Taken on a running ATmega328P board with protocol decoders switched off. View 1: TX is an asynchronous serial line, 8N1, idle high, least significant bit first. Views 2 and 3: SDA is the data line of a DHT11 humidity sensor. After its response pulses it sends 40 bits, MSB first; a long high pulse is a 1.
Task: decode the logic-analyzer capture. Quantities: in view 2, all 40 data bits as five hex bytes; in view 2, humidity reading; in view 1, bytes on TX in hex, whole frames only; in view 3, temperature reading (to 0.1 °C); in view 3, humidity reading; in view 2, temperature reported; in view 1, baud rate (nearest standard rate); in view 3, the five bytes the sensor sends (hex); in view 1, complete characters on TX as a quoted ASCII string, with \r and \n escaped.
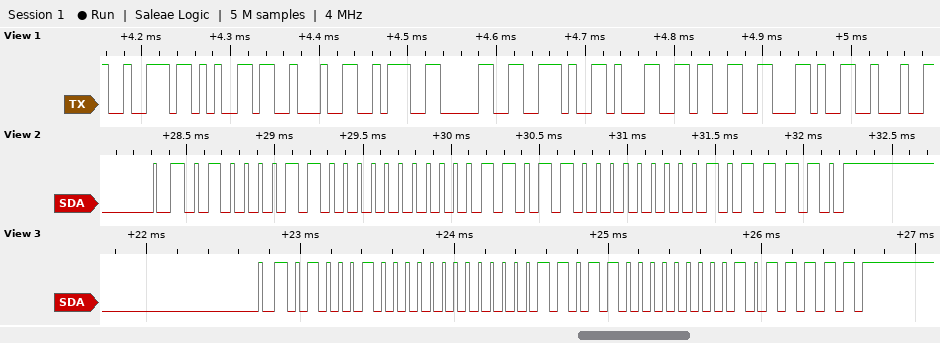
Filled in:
43 00 1B 00 5E
67 %
72 65 22 3A 30 2E 31 33 2C 22
27.0 °C
68 %
27.0 °C
115200 baud
44 00 1B 00 5F
"re\":0.13,\""
